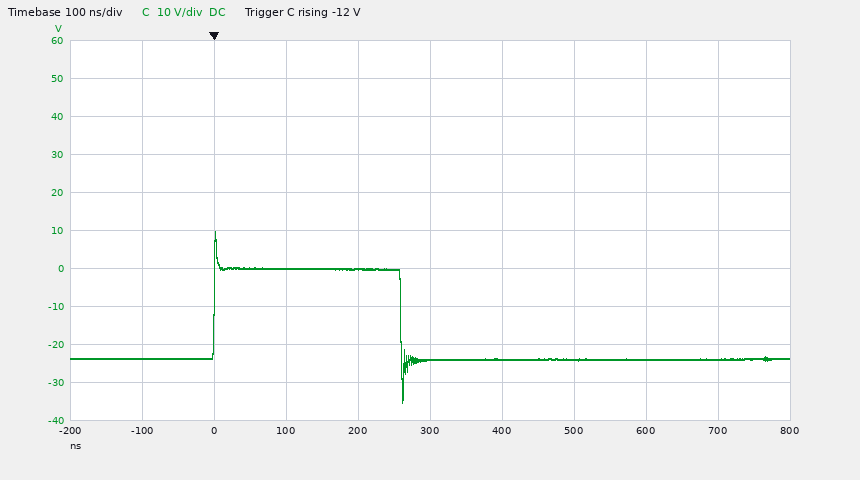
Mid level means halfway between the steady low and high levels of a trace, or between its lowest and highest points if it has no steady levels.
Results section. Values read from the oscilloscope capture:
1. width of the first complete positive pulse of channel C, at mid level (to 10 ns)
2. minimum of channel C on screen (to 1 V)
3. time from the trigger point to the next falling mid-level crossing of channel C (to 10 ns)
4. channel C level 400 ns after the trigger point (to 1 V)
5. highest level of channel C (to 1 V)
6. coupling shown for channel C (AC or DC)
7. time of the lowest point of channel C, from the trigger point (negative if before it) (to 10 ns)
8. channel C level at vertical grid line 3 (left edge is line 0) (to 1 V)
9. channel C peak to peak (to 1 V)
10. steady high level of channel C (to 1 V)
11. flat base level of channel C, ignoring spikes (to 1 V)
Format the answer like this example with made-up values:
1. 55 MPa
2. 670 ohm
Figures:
1. 260 ns
2. -35 V
3. 260 ns
4. -24 V
5. 10 V
6. DC
7. +260 ns
8. 0 V
9. 45 V
10. 0 V
11. -24 V
